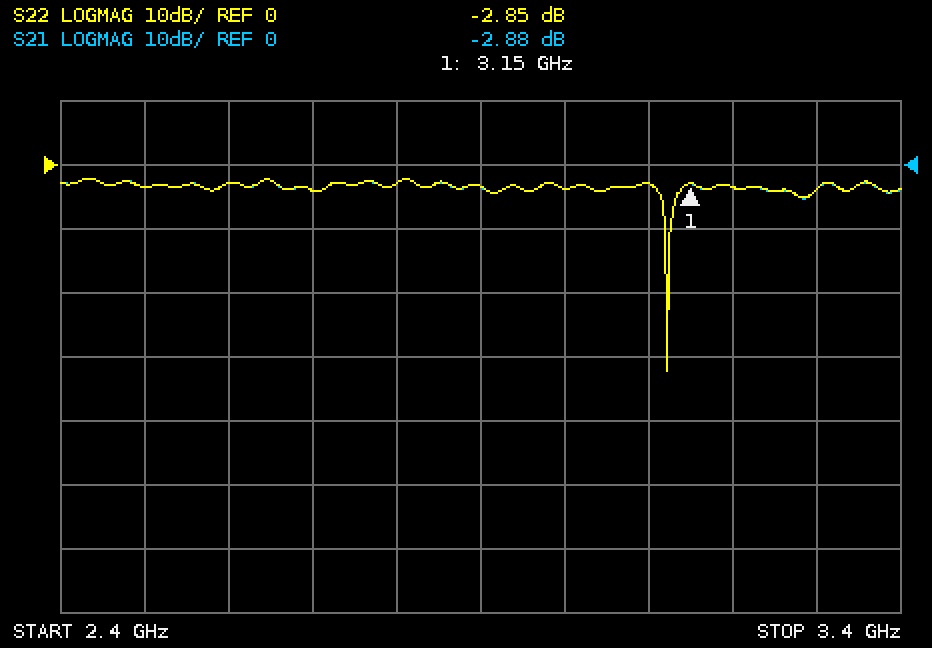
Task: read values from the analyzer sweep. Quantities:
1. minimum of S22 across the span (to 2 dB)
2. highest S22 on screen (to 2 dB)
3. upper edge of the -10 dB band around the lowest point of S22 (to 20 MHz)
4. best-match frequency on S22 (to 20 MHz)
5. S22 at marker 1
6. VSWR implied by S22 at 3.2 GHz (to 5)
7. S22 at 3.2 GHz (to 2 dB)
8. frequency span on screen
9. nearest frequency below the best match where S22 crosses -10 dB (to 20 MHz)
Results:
-32 dB
-2 dB
3.12 GHz
3.12 GHz
-2.85 dB
5
-4 dB
1 GHz
3.12 GHz
